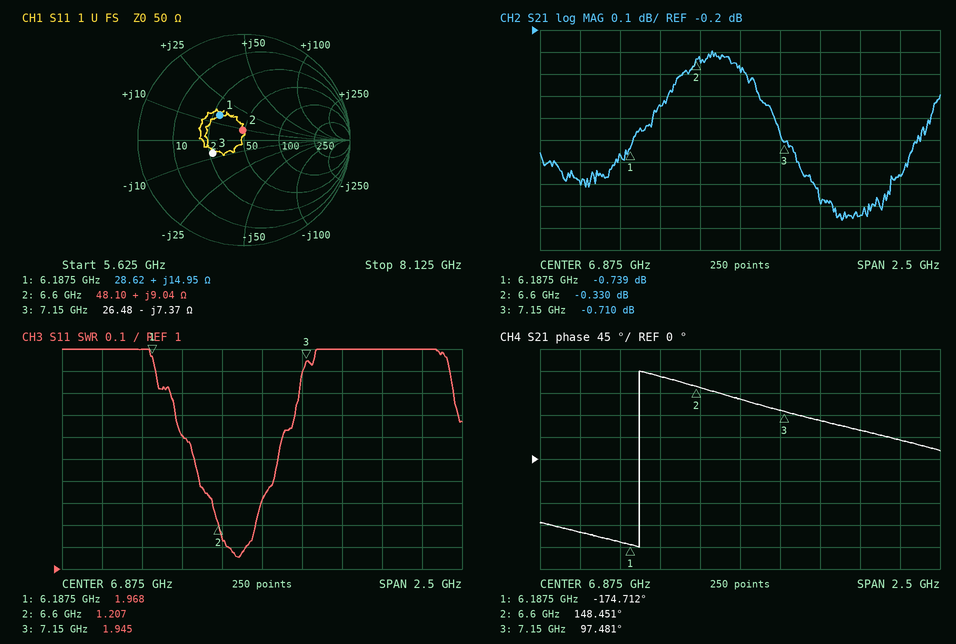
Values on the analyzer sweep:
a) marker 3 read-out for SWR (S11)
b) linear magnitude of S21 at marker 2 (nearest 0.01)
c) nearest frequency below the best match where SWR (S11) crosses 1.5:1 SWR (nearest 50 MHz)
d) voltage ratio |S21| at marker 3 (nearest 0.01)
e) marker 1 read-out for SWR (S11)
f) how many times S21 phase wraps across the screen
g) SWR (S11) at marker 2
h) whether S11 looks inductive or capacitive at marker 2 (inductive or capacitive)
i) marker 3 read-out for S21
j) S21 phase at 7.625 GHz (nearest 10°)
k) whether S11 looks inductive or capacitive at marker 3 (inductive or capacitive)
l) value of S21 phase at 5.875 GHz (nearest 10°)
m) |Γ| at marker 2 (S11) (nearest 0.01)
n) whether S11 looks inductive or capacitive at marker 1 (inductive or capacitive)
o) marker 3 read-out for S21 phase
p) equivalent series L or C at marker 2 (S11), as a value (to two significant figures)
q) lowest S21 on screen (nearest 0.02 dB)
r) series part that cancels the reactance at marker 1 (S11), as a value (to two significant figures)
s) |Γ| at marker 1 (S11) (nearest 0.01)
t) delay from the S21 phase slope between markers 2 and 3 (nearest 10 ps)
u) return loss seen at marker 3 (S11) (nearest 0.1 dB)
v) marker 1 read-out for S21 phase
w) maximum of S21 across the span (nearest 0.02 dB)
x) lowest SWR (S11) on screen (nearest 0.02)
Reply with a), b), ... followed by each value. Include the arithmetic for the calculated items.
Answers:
a) 1.945
b) 10^(-0.33/20) ≈ 0.96
c) 6.45 GHz
d) 10^(-0.71/20) ≈ 0.92
e) 1.968
f) 1
g) 1.207
h) inductive
i) -0.710 dB
j) 60°
k) capacitive
l) -150°
m) 0.09
n) inductive
o) 97.481°
p) L = 9.04 Ω/(2π × 6.6 GHz) ≈ 218 pH, so 220 pH to two significant figures
q) -1.06 dB
r) C = 1/(2π × 6.1875 GHz × 14.95 Ω) ≈ 1.7 pF
s) 0.33
t) −(97.481° − (148.451°))/(360° × 550 MHz) ≈ 257 ps, so 260 ps to the nearest 10 ps
u) 9.9 dB
v) -174.712°
w) -0.30 dB
x) 1.06
